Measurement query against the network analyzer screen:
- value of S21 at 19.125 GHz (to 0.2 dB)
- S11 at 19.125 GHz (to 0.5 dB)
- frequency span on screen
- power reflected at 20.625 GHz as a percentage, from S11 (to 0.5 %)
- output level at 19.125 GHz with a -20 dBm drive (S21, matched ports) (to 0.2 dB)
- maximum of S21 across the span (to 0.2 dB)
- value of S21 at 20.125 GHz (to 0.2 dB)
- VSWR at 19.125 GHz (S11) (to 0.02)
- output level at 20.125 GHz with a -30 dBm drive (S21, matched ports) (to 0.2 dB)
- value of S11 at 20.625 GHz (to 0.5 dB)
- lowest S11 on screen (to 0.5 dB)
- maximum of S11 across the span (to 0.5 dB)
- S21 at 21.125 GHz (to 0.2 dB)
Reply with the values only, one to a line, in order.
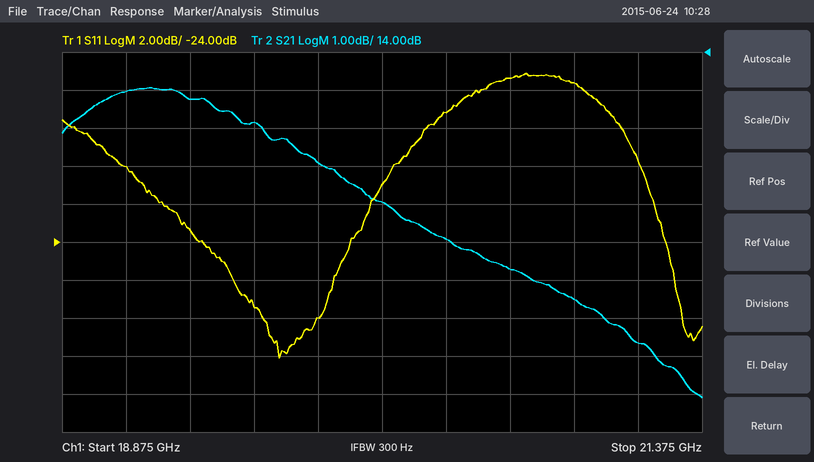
13.0 dB
-20.0 dB
2.5 GHz
3.0 %
-7.0 dBm
13.0 dB
10.0 dB
1.22
-20.0 dBm
-15.5 dB
-30.0 dB
-15.0 dB
6.4 dB
